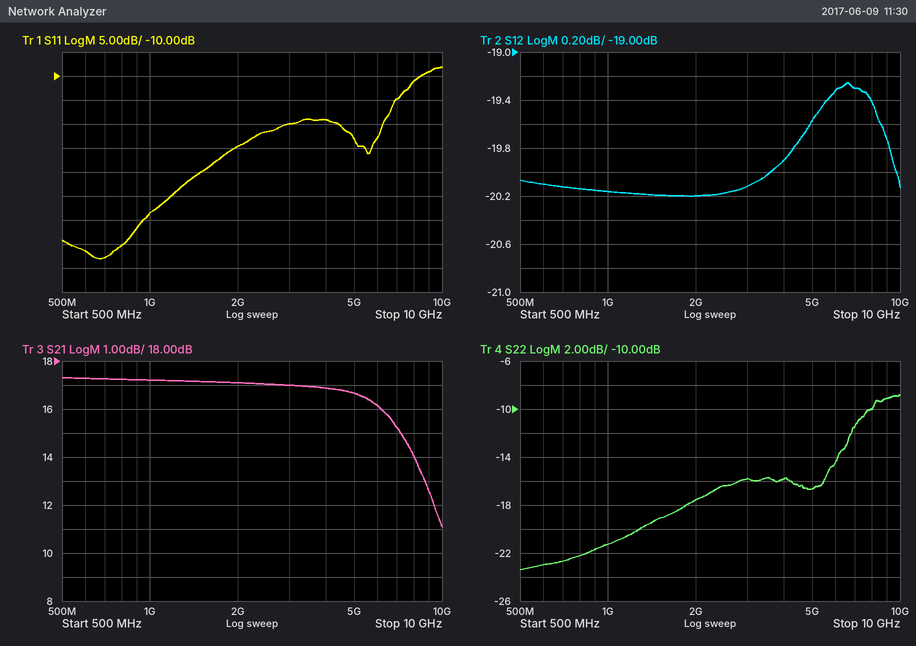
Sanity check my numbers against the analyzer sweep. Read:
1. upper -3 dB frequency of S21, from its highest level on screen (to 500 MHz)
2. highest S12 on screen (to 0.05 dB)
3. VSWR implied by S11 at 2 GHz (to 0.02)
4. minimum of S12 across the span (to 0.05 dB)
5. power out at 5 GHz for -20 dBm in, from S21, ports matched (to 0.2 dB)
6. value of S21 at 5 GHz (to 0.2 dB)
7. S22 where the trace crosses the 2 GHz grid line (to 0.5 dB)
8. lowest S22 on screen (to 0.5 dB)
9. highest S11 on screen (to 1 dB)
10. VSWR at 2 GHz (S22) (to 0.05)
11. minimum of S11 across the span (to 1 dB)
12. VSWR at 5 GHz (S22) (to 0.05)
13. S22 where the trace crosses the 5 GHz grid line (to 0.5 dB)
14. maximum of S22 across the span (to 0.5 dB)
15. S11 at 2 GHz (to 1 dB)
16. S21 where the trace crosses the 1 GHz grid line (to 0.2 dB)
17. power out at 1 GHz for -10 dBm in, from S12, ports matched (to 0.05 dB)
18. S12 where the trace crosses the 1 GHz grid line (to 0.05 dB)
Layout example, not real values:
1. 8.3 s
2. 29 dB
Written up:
1. 8.0 GHz
2. -19.25 dB
3. 1.12
4. -20.20 dB
5. -3.4 dBm
6. 16.6 dB
7. -17.5 dB
8. -23.5 dB
9. -8 dB
10. 1.30
11. -48 dB
12. 1.35
13. -16.5 dB
14. -9.0 dB
15. -25 dB
16. 17.2 dB
17. -30.15 dBm
18. -20.15 dB
